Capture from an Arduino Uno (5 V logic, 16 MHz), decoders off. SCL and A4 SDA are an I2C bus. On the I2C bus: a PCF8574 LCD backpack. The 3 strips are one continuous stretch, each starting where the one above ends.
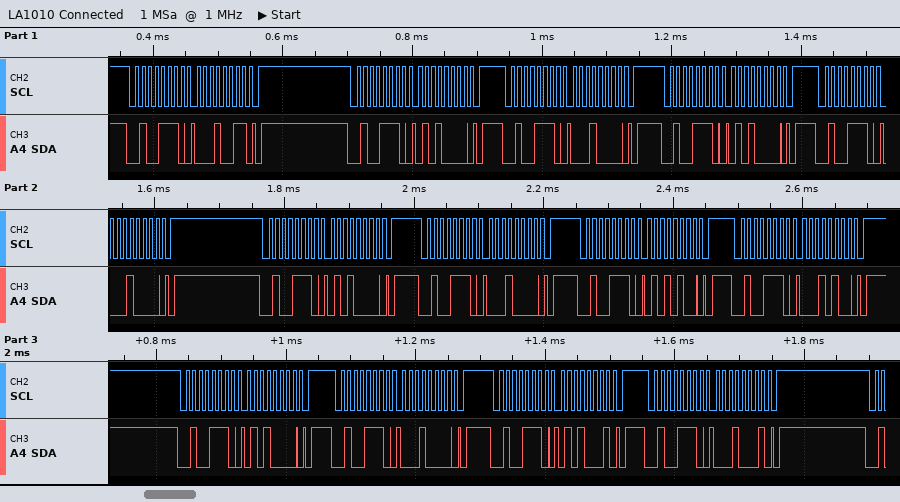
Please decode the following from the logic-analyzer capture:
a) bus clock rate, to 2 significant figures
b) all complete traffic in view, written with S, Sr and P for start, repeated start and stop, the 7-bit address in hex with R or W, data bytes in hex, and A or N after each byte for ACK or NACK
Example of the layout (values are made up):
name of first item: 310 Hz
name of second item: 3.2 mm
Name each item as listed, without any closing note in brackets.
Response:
bus clock rate, to 2 significant figures: 100 kHz
all complete traffic in view, written with S, Sr and P for start, repeated start and stop, the 7-bit address in hex with R or W, data bytes in hex, and A or N after each byte for ACK or NACK: S 27W A 13 A P S 27W A 50 A P S 27W A 10 A P S 27W A 50 A P S 27W A 10 A P S 27W A 50 A P S 27W A 10 A P S 27W A 54 A P S 27W A 14 A P S 27W A 50 A P S 27W A 10 A P S 27W A 51 A P S 27W A 11 A P
